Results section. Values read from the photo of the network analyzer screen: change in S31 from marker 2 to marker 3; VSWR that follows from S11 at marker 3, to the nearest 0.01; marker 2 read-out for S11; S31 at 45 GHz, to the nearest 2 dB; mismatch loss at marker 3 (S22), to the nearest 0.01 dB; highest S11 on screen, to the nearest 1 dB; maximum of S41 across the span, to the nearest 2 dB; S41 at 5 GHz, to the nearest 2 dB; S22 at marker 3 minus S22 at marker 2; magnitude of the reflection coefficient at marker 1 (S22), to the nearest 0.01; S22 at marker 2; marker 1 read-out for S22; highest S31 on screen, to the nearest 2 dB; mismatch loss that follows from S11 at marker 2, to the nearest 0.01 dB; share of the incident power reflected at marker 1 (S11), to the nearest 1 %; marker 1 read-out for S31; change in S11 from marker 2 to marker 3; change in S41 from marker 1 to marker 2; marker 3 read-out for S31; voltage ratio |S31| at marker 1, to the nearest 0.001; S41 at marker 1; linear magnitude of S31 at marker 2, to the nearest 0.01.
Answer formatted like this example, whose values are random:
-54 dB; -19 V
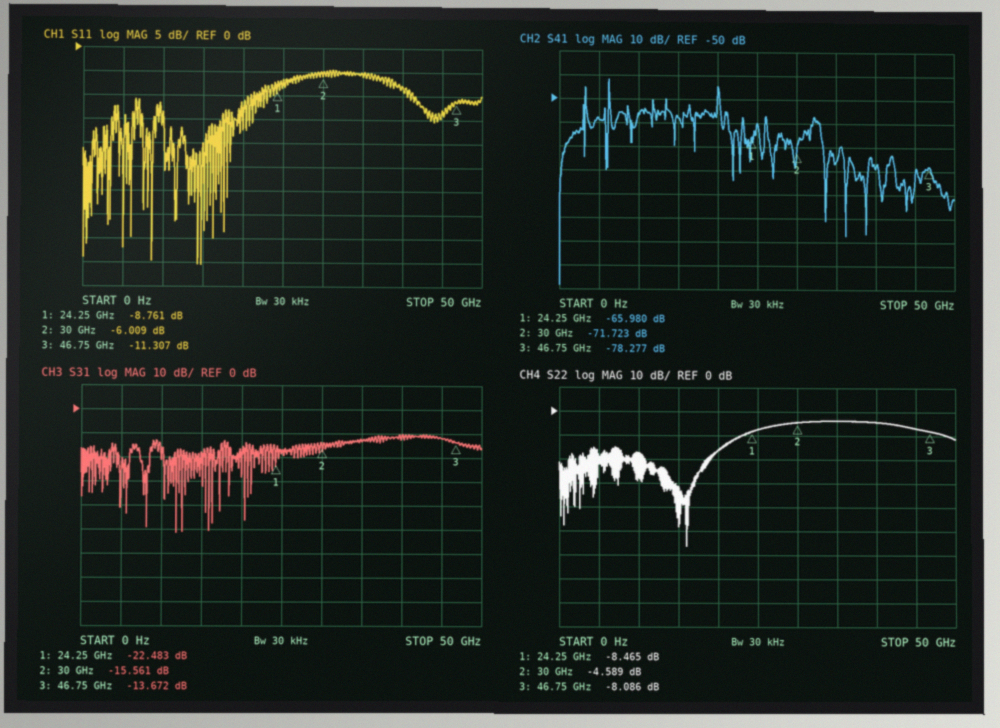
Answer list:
1.889 dB; 1.75; -6.009 dB; -12 dB; 0.73 dB; -5 dB; -42 dB; -58 dB; -3.497 dB; 0.38; -4.589 dB; -8.465 dB; -10 dB; 1.25 dB; 13 %; -22.483 dB; -5.298 dB; -5.743 dB; -13.672 dB; 0.075; -65.980 dB; 0.17
